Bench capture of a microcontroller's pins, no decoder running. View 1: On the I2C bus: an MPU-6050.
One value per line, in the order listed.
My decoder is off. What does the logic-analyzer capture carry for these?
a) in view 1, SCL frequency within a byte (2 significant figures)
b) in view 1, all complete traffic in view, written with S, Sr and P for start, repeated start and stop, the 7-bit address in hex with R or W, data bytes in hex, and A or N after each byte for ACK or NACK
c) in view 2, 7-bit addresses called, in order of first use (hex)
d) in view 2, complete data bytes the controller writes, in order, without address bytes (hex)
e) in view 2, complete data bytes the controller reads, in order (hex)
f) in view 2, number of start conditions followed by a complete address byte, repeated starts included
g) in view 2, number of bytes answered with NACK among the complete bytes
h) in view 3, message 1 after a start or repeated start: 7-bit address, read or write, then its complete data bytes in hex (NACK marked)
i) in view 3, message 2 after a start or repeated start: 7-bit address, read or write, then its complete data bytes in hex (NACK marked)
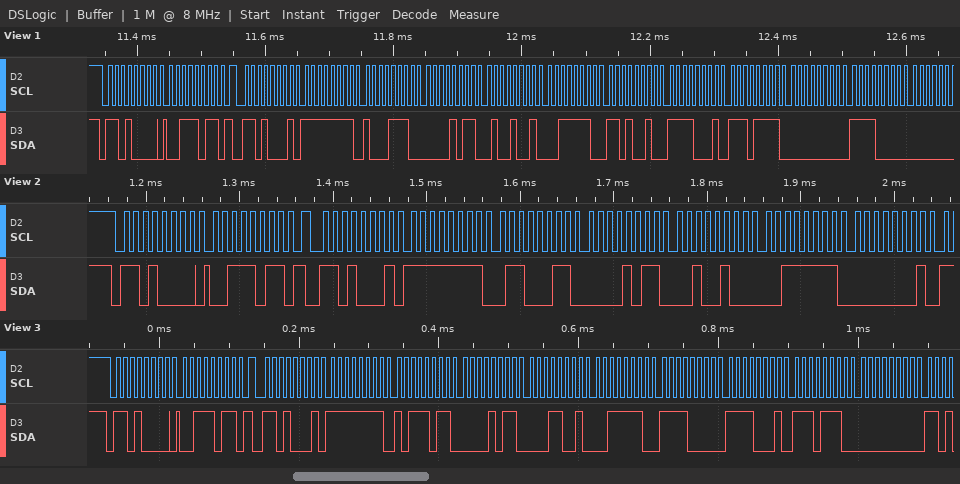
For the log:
100 kHz
S 68W A 3B A Sr 68R A FF A 8E A 0B A 49 A 3E A D2 A F1 A EF A 00 A F0 A
0x68
3B
FF 63 0B 24 3F 01
2
0
0x68 write: 3B
0x68 read: FF BB 0B 19 3E F0 F1 EE 00
